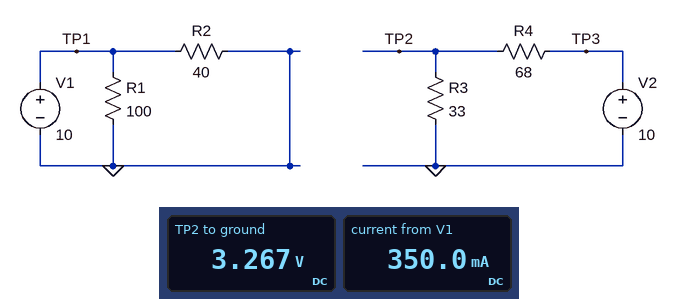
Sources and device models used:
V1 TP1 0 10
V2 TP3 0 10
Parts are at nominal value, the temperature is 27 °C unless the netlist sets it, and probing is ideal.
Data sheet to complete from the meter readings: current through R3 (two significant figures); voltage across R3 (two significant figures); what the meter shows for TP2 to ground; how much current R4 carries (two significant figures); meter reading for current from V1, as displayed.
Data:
99 mA
3.3 V
3.267 V
99 mA
350.0 mA
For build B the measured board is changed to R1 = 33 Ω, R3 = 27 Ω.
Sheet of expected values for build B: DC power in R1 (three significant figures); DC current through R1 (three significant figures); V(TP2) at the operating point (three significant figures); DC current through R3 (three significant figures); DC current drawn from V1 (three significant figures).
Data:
3.03 W
303 mA
2.84 V
105 mA
553 mA
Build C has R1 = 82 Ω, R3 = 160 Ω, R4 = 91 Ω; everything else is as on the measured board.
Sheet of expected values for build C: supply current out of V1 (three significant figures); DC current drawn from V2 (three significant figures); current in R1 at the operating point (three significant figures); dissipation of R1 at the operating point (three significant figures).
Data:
372 mA
39.8 mA
122 mA
1.22 W
